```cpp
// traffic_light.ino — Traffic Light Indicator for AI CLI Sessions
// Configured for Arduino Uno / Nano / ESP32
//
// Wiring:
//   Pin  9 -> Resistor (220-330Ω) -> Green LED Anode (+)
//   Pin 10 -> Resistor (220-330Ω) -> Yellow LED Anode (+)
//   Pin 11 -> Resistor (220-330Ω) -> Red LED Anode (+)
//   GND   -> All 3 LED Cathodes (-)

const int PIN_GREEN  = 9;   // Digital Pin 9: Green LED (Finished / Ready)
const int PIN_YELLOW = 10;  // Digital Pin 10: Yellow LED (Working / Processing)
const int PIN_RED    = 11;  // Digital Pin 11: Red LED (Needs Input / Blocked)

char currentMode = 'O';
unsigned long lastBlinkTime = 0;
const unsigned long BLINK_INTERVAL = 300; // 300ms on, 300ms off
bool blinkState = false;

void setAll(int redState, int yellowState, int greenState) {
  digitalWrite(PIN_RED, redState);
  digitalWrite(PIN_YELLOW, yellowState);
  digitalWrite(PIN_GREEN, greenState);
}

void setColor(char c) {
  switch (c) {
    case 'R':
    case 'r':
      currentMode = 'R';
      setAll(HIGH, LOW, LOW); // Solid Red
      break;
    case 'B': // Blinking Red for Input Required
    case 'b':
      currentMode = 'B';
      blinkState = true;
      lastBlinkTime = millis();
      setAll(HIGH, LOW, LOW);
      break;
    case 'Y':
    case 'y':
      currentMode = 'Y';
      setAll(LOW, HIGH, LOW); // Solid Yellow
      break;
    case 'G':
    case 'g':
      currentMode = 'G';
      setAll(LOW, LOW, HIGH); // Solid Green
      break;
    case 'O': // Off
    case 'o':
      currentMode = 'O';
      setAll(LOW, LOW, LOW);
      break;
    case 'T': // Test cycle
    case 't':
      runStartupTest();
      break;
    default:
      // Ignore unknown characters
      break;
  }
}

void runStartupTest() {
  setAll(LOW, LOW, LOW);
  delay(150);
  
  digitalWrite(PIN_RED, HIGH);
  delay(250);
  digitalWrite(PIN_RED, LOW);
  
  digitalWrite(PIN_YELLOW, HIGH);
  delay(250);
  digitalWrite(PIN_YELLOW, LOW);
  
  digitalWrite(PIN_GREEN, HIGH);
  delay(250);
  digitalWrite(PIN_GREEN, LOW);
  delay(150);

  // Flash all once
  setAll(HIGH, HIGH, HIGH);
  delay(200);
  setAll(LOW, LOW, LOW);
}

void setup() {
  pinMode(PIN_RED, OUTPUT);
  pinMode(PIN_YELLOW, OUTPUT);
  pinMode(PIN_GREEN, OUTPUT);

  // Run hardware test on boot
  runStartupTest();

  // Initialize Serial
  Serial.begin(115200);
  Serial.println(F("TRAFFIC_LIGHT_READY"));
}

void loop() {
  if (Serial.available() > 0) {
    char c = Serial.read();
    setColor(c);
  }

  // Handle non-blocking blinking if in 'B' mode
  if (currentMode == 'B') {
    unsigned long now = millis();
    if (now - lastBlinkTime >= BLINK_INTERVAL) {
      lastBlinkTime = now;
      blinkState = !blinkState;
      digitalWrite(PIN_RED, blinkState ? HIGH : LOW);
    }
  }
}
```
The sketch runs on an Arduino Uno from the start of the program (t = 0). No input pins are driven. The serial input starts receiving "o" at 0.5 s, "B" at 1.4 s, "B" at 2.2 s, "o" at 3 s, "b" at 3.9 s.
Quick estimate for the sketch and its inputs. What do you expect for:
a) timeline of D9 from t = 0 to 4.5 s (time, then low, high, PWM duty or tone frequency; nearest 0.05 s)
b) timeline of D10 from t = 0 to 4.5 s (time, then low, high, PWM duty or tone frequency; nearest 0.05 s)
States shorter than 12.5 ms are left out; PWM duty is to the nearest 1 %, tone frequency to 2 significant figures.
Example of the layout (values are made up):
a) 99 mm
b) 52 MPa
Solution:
a) 0 s low; 0.65 s high; 0.9 s low; 1.05 s high; 1.25 s low
b) 0 s low; 0.4 s high; 0.65 s low; 1.05 s high; 1.25 s low
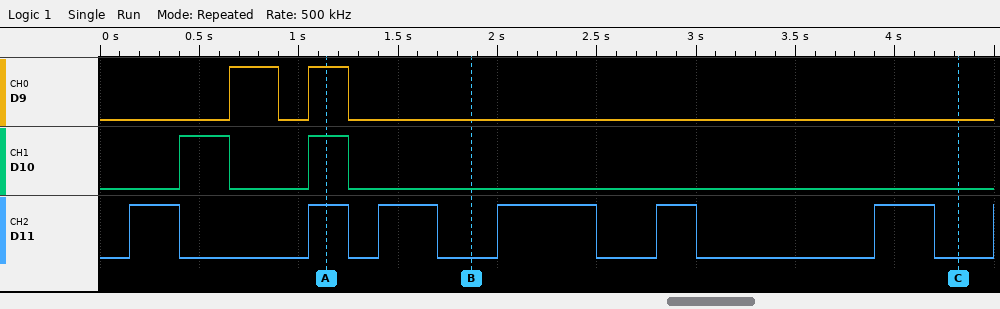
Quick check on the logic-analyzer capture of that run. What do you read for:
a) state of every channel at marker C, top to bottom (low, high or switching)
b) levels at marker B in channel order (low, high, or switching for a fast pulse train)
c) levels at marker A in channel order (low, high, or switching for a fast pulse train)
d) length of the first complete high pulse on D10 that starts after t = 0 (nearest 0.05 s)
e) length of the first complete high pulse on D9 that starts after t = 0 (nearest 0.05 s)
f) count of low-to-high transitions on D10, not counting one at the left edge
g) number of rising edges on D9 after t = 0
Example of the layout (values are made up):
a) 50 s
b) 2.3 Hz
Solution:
a) D9 low, D10 low, D11 low
b) D9 low, D10 low, D11 low
c) D9 high, D10 high, D11 high
d) 0.25 s
e) 0.25 s
f) 2
g) 2
